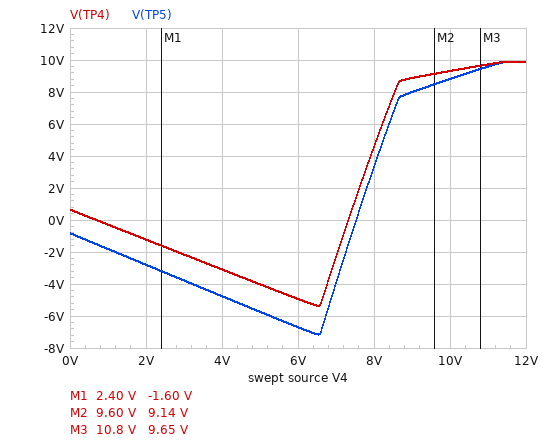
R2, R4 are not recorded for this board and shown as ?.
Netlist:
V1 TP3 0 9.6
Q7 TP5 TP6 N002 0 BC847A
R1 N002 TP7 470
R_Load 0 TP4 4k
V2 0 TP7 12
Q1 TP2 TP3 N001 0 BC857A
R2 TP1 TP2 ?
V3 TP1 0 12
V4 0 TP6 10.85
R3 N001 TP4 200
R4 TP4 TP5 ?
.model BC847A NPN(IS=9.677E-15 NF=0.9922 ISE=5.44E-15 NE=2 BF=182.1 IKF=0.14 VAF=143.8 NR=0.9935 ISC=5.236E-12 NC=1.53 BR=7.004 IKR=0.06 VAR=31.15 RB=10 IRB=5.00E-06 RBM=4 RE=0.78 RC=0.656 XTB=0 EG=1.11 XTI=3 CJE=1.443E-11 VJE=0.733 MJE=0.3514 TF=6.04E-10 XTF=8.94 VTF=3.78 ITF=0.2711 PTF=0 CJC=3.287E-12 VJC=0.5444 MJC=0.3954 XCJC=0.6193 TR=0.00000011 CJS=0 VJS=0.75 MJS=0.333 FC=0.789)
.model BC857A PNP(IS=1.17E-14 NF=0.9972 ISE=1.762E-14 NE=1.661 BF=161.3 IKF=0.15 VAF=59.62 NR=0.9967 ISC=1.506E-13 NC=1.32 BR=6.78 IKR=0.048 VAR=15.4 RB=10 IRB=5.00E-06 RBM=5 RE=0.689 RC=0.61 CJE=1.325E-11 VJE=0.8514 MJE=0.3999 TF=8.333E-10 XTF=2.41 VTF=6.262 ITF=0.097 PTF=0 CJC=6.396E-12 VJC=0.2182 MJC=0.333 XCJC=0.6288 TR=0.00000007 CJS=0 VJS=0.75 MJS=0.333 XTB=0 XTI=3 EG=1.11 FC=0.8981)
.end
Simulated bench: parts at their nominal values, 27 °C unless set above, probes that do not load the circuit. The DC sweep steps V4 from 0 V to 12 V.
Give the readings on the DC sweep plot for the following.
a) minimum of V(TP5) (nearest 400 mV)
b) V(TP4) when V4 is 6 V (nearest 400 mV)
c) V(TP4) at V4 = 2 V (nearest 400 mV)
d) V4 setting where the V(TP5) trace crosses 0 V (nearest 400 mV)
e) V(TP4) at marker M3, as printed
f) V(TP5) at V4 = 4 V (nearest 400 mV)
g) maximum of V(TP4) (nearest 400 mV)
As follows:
-7.2 V
-4.8 V
-1.2 V
7.6 V
9.65 V
-4.8 V
10.0 V
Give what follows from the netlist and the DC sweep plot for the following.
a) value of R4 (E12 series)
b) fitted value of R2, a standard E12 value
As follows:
180 Ω
180 Ω
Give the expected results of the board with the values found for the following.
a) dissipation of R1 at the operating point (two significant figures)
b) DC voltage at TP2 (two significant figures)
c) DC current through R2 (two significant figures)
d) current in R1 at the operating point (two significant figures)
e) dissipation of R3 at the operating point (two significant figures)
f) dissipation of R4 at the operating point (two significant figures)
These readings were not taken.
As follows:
530 µW
10 V
9.0 mA
1.1 mA
2.4 mW
200 µW
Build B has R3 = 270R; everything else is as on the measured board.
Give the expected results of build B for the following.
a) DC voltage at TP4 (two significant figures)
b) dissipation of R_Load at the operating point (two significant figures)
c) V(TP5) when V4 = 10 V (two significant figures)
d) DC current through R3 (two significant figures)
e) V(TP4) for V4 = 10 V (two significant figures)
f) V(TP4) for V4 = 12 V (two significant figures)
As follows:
9.4 V
22 mW
8.5 V
3.4 mA
9.0 V
9.7 V
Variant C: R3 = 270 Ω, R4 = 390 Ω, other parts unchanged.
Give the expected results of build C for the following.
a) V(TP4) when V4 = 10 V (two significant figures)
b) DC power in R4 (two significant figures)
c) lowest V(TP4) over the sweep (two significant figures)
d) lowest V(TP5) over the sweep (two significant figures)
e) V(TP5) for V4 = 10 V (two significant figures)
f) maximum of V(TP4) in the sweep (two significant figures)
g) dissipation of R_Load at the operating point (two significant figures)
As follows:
9.0 V
440 µW
-3.7 V
-7.4 V
7.9 V
9.7 V
22 mW
